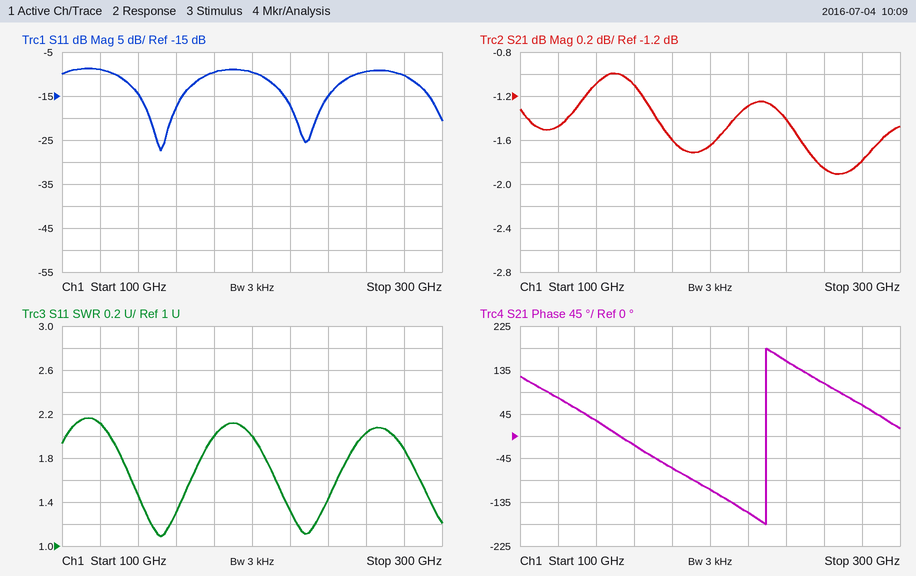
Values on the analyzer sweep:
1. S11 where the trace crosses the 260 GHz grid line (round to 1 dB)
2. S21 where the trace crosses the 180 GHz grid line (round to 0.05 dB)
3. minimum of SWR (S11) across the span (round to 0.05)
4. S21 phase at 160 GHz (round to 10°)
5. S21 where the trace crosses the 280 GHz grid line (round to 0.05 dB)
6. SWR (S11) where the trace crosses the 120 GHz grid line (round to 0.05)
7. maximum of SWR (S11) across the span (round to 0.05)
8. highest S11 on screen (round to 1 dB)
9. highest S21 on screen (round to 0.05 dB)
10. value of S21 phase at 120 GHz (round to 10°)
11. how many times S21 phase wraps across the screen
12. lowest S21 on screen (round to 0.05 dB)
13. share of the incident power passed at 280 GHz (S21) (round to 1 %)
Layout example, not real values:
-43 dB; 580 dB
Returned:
-9 dB; -1.60 dB; 1.10; -20°; -1.80 dB; 2.10; 2.15; -9 dB; -1.00 dB; 80°; 1; -1.90 dB; 66 %
